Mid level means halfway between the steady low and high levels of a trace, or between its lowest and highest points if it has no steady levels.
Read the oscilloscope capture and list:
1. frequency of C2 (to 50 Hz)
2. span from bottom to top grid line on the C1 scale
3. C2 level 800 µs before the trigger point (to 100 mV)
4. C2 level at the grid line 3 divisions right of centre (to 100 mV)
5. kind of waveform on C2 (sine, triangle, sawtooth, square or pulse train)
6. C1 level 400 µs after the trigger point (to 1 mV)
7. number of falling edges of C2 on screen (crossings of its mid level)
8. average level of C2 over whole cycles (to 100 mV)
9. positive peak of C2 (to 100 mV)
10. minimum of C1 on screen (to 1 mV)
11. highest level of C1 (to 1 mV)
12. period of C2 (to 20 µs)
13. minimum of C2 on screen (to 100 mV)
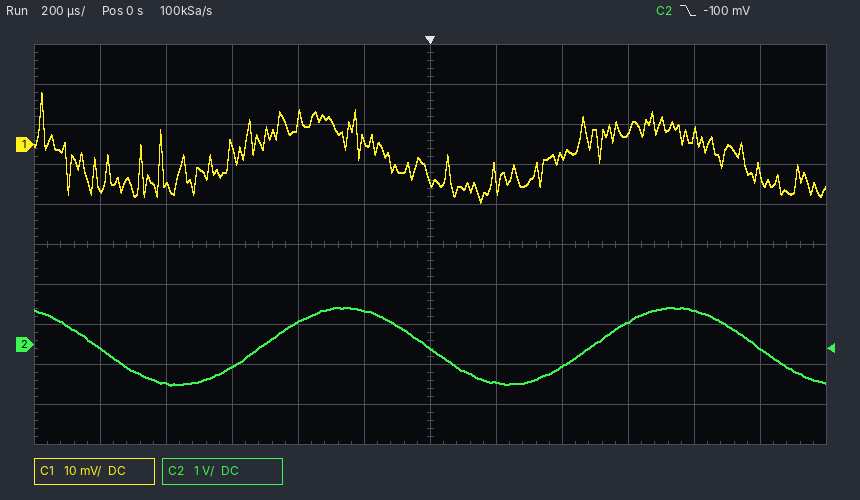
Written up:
1.00 kHz
100 mV
-1.0 V
600 mV
sine
-3 mV
3
0.0 V
900 mV
-14 mV
13 mV
1.00 ms
-1.0 V
